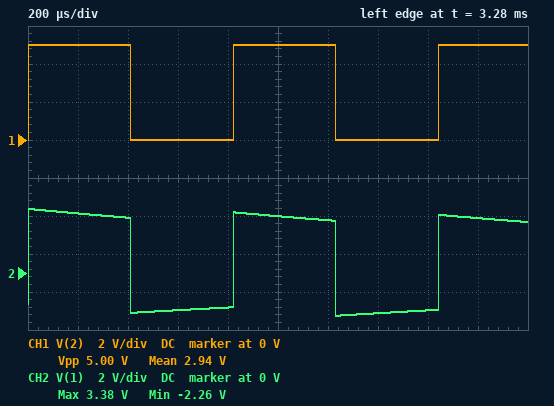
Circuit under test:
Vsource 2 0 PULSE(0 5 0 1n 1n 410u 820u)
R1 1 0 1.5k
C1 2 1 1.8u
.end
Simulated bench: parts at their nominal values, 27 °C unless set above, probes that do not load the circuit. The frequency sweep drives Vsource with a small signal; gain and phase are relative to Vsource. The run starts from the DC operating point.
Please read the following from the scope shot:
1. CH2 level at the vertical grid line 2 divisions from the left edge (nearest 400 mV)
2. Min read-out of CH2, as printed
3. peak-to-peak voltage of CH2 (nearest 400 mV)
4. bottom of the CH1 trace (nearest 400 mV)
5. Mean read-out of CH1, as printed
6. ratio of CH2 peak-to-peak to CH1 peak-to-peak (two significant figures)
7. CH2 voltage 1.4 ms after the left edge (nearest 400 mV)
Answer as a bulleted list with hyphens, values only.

- 2.8 V
- -2.26 V
- 5.6 V
- 0 V
- 2.94 V
- 1.1
- -2.0 V
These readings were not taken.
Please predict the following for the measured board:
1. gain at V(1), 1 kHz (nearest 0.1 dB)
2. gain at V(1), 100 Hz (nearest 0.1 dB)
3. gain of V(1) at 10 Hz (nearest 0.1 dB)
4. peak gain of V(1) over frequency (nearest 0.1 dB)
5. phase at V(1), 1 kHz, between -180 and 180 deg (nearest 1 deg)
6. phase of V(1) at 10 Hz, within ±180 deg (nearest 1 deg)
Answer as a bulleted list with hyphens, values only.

- 0 dB
- -1.3 dB
- -15.5 dB
- 0 dB
- 3 deg
- 80 deg
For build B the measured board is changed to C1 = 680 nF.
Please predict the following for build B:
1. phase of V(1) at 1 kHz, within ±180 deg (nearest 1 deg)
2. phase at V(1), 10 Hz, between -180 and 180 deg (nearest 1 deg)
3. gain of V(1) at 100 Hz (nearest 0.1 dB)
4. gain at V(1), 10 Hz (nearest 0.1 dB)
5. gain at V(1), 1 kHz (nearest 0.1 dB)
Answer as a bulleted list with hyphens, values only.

- 9 deg
- 86 deg
- -5.4 dB
- -23.9 dB
- -0.1 dB
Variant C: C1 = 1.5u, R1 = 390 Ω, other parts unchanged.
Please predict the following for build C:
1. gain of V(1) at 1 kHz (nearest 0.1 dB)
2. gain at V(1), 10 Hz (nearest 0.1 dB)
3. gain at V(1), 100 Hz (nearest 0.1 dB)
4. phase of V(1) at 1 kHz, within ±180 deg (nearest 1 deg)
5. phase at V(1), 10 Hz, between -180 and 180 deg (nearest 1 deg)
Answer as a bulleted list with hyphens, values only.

- -0.3 dB
- -28.7 dB
- -9.2 dB
- 15 deg
- 88 deg
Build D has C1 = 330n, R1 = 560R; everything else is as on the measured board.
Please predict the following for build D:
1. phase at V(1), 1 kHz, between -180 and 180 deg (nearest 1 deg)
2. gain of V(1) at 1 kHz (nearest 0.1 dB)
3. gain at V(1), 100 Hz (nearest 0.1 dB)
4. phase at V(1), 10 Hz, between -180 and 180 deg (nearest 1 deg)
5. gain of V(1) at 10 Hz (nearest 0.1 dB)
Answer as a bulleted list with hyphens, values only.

- 41 deg
- -2.4 dB
- -18.8 dB
- 89 deg
- -38.7 dB
